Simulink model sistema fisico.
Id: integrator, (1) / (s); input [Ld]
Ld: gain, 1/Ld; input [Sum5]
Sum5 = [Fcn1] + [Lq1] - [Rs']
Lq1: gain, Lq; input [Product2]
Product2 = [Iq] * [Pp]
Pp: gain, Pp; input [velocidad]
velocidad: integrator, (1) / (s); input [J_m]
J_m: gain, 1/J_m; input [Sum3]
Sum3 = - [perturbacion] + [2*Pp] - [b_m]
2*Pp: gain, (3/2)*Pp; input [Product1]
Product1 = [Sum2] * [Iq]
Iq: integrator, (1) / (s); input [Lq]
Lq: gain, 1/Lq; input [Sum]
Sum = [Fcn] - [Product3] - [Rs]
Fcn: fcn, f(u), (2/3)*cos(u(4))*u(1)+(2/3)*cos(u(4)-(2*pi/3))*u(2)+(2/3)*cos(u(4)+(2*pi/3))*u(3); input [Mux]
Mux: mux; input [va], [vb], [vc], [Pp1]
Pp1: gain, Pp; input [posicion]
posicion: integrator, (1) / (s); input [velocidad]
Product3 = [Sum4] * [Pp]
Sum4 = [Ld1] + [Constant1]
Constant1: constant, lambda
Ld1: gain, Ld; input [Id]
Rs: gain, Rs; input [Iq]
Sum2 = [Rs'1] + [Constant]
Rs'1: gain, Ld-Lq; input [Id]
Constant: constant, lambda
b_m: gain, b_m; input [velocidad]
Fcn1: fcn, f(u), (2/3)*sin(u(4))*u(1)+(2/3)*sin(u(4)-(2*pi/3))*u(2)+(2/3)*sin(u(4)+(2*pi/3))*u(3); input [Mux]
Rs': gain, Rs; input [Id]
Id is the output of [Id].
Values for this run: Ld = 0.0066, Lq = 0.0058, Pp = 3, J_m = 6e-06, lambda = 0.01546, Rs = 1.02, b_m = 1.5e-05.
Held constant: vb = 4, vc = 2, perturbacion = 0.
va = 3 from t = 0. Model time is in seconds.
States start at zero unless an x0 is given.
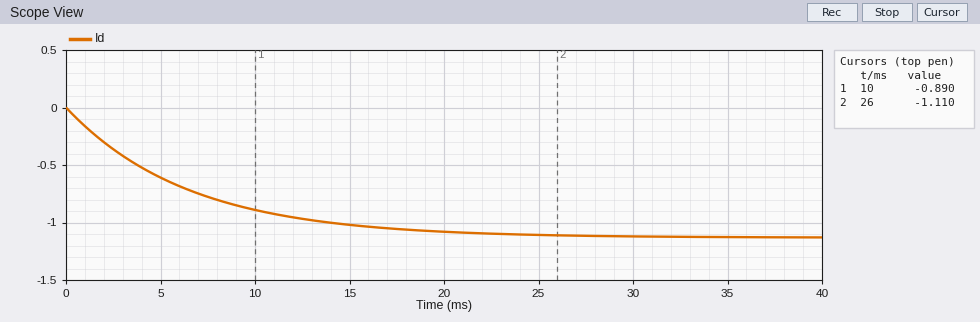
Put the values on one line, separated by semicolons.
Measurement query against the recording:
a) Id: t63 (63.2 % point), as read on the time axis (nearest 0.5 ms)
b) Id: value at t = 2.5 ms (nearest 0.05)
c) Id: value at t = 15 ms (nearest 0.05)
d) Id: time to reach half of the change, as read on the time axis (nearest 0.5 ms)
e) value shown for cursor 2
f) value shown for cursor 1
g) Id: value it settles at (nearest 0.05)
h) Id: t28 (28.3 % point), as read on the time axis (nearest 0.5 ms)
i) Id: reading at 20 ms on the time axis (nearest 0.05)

6.5 ms; -0.35; -1.00; 4.5 ms; -1.110; -0.890; -1.15; 2.0 ms; -1.10
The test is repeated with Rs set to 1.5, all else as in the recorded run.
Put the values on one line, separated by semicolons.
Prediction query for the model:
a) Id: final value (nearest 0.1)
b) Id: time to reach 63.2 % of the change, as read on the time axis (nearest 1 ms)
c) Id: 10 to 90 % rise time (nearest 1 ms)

-0.8; 4 ms; 10 ms
